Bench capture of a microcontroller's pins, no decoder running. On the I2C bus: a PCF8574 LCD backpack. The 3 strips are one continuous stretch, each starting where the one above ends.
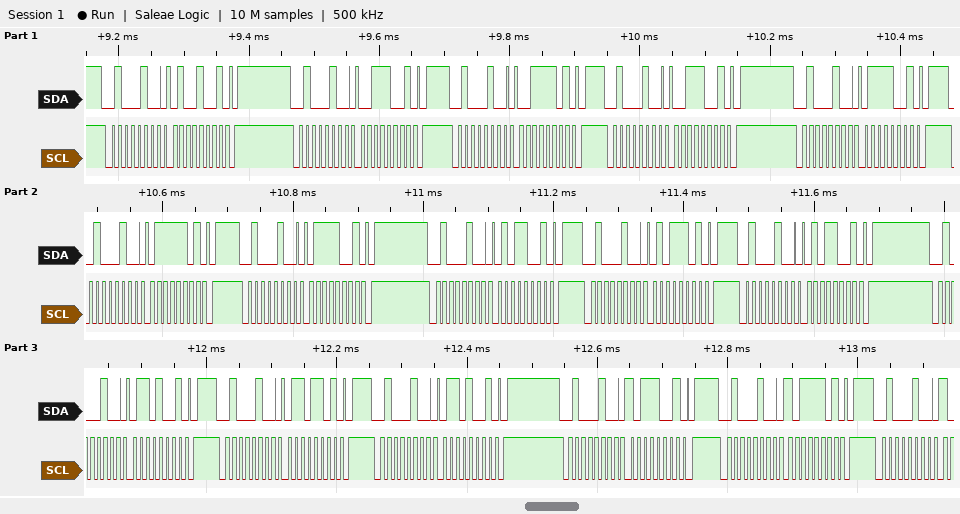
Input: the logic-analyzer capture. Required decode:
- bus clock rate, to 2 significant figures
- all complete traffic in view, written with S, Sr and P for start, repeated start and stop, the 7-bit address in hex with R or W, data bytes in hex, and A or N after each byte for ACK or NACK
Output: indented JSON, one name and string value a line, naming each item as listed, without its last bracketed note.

{
  "bus clock rate, to 2 significant figures": "100 kHz",
  "all complete traffic in view, written with S, Sr and P for start, repeated start and stop, the 7-bit address in hex with R or W, data bytes in hex, and A or N after each byte for ACK or NACK": "S 22W A 49 A P S 22W A 39 A P S 22W A 3D A P S 22W A 39 A P S 22W A 79 A P S 22W A 7D A P S 22W A 79 A P S 22W A 59 A P S 22W A 5D A P S 22W A 59 A P S 22W A 69 A P S 22W A 6D A P S 22W A 69 A P S 22W A B9 A P S 22W A BD A P S 22W A"
}
